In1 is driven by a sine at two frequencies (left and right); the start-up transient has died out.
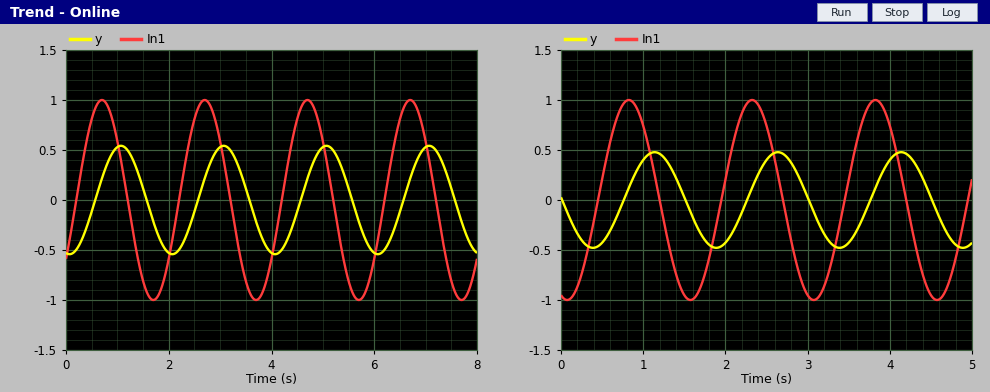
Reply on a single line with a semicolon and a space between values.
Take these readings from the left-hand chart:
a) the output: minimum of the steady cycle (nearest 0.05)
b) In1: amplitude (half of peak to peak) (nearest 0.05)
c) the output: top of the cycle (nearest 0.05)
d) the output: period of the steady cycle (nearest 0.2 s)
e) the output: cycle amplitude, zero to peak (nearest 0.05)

-0.55; 1.00; 0.55; 2.0 s; 0.55
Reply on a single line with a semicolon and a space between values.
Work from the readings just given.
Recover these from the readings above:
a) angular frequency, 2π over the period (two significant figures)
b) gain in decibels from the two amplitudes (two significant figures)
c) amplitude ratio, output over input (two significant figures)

3.1 rad/s; -5.2 dB; 0.55
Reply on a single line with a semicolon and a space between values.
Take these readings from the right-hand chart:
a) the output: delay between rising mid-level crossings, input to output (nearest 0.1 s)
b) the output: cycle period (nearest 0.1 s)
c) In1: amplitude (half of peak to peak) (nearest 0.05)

0.3 s; 1.5 s; 1.00
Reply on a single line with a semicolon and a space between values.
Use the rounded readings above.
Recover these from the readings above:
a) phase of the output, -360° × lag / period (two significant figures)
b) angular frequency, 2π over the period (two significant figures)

-72°; 4.2 rad/s
